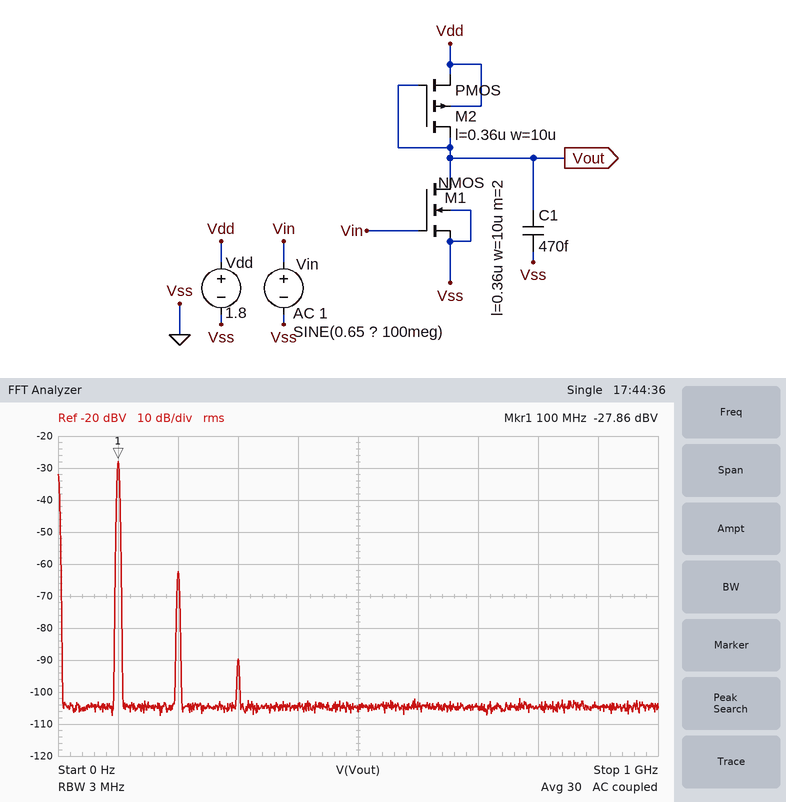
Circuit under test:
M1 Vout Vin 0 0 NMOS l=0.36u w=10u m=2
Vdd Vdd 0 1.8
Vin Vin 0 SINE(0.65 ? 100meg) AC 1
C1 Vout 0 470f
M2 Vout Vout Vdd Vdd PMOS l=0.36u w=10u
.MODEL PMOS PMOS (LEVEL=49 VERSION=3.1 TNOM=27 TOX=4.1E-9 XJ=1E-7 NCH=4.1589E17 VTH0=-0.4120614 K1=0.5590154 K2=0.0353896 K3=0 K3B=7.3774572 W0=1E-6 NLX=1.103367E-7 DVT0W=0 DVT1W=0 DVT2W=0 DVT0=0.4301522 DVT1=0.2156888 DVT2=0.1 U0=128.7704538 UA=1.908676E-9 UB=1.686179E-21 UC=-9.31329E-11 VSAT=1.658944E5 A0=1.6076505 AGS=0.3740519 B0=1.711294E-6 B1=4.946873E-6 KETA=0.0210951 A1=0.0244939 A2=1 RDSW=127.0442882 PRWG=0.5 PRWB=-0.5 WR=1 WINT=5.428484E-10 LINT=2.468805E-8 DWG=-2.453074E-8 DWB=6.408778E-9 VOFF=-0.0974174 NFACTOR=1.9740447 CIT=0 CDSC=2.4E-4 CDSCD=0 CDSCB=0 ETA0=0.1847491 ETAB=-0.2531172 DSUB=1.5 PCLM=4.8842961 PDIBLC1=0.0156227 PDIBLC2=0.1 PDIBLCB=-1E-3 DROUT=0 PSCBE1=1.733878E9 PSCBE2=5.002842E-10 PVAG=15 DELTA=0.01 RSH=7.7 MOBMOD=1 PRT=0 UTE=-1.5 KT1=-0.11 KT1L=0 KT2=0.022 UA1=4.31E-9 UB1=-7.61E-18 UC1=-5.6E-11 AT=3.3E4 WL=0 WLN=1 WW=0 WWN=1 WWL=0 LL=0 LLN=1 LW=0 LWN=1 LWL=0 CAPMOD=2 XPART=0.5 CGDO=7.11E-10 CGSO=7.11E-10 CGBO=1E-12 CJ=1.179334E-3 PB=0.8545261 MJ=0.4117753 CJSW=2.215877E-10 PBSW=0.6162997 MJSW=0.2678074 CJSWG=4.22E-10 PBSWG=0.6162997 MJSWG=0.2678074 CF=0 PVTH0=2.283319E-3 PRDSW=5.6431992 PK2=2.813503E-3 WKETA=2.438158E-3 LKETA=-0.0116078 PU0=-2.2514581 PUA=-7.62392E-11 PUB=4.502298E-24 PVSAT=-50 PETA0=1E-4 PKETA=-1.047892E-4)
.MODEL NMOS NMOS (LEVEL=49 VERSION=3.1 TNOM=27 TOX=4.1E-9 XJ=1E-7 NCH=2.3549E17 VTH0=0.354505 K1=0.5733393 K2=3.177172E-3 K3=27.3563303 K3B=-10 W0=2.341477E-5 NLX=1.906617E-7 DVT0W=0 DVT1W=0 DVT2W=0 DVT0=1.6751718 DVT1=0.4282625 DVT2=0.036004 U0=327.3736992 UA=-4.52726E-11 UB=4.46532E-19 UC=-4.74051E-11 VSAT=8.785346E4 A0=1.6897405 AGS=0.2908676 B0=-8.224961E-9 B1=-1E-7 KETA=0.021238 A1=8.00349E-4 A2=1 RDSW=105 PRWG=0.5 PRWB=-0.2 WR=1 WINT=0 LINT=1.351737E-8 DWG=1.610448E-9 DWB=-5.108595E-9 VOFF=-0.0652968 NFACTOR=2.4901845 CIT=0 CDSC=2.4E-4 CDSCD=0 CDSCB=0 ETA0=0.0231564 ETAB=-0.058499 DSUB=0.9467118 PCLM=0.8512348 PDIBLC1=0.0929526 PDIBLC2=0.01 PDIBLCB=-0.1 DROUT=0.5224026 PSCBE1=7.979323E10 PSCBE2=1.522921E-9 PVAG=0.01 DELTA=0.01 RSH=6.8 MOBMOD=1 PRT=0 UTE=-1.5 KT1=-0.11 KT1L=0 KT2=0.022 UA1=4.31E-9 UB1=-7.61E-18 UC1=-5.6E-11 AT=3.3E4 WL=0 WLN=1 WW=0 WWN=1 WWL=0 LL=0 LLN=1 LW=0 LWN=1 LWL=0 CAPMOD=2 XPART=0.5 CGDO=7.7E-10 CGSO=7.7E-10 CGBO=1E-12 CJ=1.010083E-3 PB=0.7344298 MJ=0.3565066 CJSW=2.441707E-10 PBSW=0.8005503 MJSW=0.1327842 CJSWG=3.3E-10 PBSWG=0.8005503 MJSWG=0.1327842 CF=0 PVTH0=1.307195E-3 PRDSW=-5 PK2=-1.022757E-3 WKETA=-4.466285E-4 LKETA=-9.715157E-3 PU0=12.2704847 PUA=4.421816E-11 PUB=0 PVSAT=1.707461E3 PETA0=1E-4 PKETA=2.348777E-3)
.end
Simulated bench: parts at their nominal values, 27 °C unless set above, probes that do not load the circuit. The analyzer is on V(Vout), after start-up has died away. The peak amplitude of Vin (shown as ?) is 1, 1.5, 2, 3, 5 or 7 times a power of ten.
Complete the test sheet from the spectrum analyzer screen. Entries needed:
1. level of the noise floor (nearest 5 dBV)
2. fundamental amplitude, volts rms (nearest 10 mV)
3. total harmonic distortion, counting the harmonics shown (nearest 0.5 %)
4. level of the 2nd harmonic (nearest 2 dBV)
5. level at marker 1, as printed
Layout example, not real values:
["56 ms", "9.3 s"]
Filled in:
["-105 dBV", "40 mV", "2.0 %", "-62 dBV", "-27.86 dBV"]
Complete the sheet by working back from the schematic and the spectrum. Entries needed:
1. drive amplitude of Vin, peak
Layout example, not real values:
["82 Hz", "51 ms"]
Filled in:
["20 mV"]
